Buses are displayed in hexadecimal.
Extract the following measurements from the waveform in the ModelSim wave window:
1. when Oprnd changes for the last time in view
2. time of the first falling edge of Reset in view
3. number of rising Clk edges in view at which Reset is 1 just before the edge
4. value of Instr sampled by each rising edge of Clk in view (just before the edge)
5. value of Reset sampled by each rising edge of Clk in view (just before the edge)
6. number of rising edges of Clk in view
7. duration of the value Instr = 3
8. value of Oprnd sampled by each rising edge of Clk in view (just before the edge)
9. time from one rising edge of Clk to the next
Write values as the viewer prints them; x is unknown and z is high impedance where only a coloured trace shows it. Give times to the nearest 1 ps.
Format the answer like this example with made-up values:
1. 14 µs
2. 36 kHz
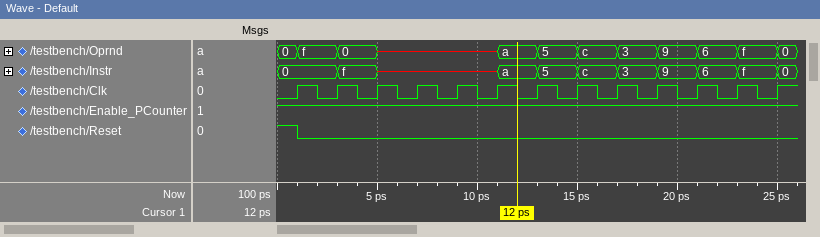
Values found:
1. 25 ps
2. 1 ps
3. 1
4. 0, 0, f, x, x, x, a, 5, c, 3, 9, 6, f
5. 1 0 0 0 0 0 0 0 0 0 0 0 0
6. 13
7. 2 ps
8. 0, f, 0, x, x, x, a, 5, c, 3, 9, 6, f
9. 2 ps
